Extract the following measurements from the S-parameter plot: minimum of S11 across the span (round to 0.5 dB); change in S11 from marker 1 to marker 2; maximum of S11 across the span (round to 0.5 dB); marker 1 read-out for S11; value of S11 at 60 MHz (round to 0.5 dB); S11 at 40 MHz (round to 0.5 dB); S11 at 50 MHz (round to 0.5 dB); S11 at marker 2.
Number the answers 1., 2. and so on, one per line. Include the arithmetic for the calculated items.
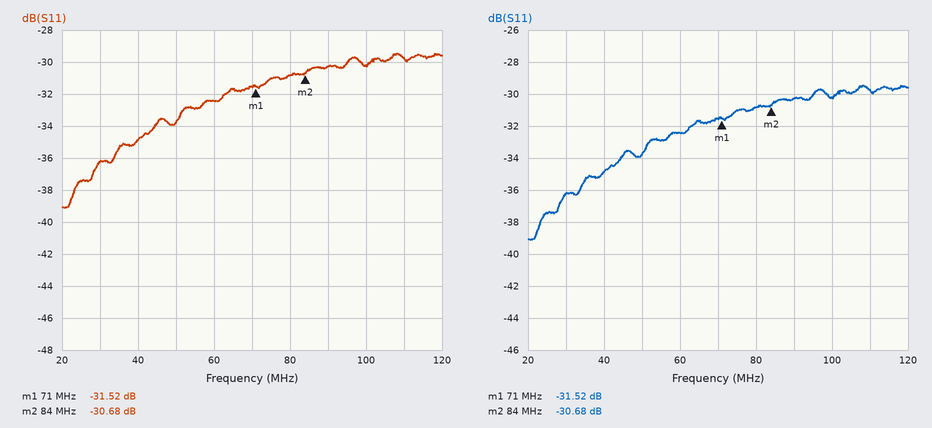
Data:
1. -39.0 dB
2. -30.68 − (-31.52) = 0.84 dB
3. -29.5 dB
4. -31.52 dB
5. -32.5 dB
6. -35.0 dB
7. -34.0 dB
8. -30.68 dB
